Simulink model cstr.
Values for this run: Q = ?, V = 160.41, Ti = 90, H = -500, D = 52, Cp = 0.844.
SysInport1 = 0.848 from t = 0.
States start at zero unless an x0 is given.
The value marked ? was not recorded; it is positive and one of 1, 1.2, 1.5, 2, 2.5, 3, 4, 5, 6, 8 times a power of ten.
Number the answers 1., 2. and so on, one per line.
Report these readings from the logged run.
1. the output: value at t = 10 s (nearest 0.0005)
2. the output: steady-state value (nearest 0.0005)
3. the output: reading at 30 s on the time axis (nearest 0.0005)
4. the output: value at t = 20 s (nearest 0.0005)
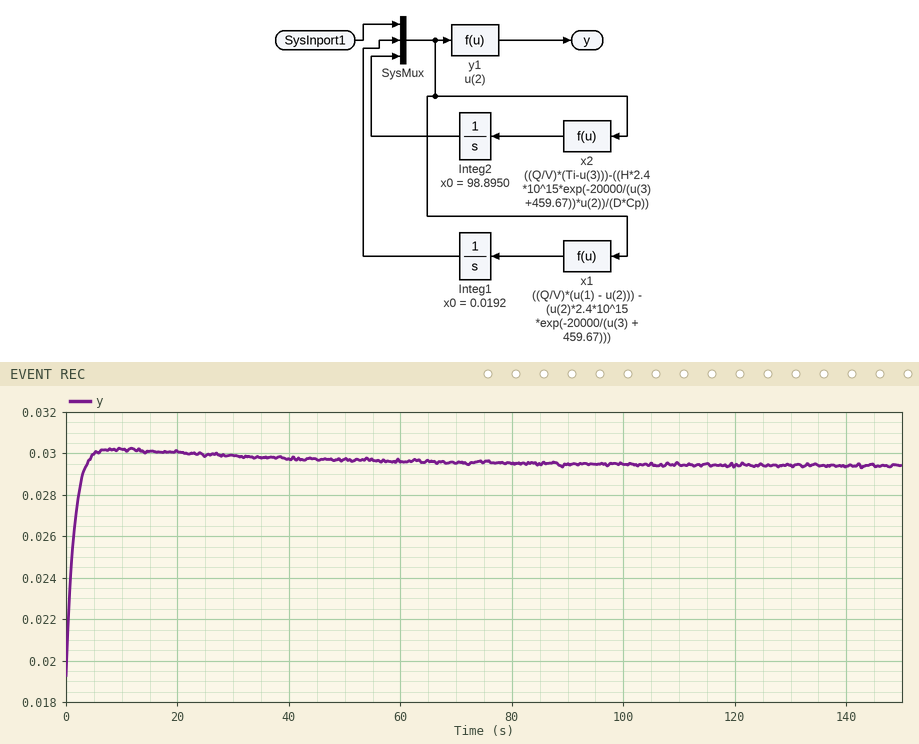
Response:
1. 0.0300
2. 0.0295
3. 0.0300
4. 0.0300
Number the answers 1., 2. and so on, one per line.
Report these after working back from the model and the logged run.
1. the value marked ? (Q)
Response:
1. 4
